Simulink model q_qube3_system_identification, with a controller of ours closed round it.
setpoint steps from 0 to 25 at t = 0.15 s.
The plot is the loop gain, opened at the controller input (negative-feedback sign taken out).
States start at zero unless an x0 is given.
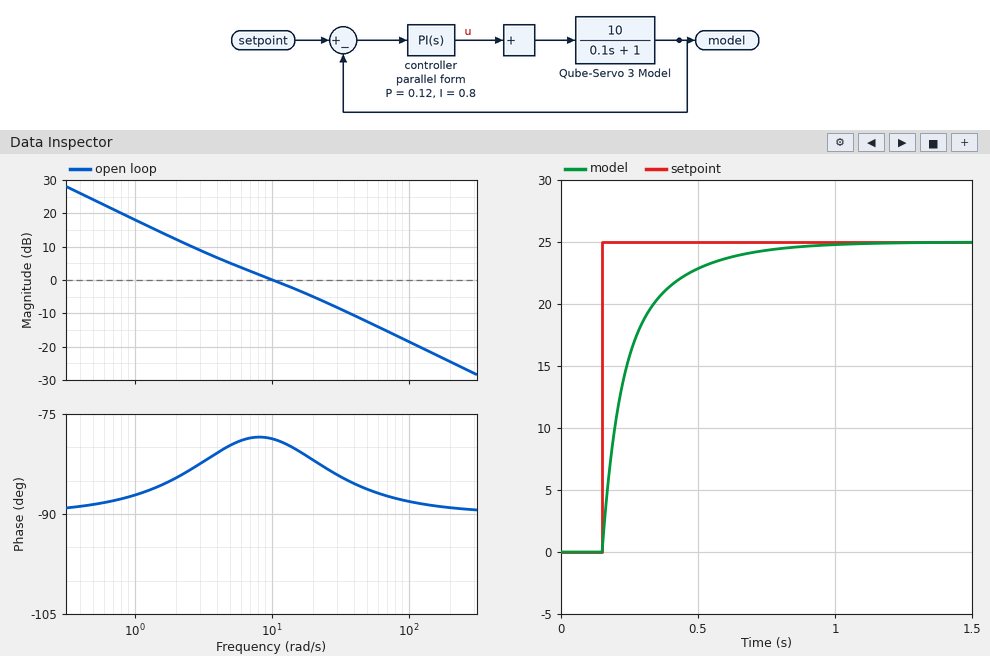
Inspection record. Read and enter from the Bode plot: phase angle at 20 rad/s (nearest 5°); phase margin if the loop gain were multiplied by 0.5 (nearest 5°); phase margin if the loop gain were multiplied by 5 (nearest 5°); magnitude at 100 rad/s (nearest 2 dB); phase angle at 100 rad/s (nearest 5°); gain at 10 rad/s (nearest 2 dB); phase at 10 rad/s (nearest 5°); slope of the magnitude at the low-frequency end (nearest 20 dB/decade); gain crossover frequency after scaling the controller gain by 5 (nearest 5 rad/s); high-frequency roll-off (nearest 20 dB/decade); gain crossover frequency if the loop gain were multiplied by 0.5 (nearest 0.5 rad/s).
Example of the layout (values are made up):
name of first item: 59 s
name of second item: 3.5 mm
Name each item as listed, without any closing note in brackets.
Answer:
phase angle at 20 rad/s: -80°
phase margin if the loop gain were multiplied by 0.5: 100°
phase margin if the loop gain were multiplied by 5: 95°
magnitude at 100 rad/s: -18 dB
phase angle at 100 rad/s: -90°
gain at 10 rad/s: 0 dB
phase at 10 rad/s: -80°
slope of the magnitude at the low-frequency end: -20 dB/decade
gain crossover frequency after scaling the controller gain by 5: 60 rad/s
high-frequency roll-off: -20 dB/decade
gain crossover frequency if the loop gain were multiplied by 0.5: 4.5 rad/s
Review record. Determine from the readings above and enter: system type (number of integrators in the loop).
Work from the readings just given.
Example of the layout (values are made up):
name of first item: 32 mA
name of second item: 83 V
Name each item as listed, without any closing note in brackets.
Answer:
system type: 1
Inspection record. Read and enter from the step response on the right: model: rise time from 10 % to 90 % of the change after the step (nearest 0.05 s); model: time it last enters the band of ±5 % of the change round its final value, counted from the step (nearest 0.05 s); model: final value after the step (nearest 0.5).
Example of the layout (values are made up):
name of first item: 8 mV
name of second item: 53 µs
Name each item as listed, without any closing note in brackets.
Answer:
model: rise time from 10 % to 90 % of the change after the step: 0.30 s
model: time it last enters the band of ±5 % of the change round its final value, counted from the step: 0.45 s
model: final value after the step: 25.0
